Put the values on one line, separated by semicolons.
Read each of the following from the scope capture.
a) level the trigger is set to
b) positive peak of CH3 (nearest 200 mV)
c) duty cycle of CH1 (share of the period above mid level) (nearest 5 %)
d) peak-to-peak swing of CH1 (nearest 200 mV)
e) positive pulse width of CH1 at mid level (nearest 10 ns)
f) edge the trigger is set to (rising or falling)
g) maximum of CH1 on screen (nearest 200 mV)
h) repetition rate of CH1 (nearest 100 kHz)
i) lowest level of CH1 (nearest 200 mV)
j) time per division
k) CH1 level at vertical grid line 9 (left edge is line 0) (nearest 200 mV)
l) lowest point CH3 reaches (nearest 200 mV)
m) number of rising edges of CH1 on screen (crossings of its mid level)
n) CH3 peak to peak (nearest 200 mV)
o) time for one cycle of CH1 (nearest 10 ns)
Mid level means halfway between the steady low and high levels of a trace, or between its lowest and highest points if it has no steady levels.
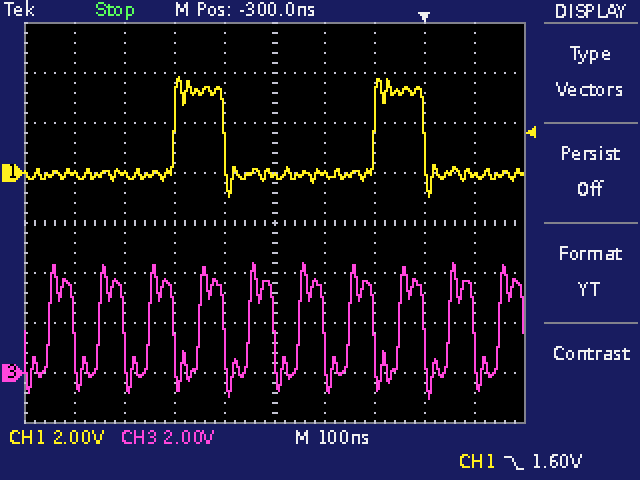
1.60 V; 4.4 V; 25 %; 4.8 V; 100 ns; falling; 3.8 V; 2.5 MHz; -1.0 V; 100 ns; 0.0 V; -1.0 V; 2; 5.4 V; 400 ns
